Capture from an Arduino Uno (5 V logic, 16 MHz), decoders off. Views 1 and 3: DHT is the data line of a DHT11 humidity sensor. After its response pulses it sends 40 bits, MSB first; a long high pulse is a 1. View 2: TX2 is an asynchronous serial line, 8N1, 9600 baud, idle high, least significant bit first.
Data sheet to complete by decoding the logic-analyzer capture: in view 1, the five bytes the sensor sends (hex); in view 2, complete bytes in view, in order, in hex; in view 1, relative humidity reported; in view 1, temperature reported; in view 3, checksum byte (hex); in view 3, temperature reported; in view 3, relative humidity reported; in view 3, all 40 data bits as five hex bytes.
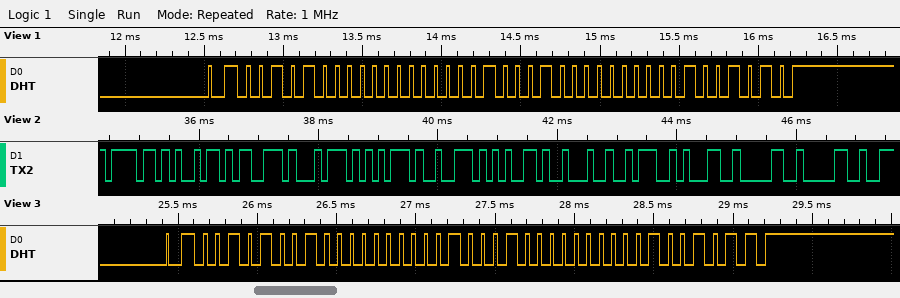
28 00 22 00 4A
6F 69 73 74 75 72 65 22 3A 31 30 30
40 %
34.0 °C
0x4B
34.0 °C
41 %
29 00 22 00 4B
